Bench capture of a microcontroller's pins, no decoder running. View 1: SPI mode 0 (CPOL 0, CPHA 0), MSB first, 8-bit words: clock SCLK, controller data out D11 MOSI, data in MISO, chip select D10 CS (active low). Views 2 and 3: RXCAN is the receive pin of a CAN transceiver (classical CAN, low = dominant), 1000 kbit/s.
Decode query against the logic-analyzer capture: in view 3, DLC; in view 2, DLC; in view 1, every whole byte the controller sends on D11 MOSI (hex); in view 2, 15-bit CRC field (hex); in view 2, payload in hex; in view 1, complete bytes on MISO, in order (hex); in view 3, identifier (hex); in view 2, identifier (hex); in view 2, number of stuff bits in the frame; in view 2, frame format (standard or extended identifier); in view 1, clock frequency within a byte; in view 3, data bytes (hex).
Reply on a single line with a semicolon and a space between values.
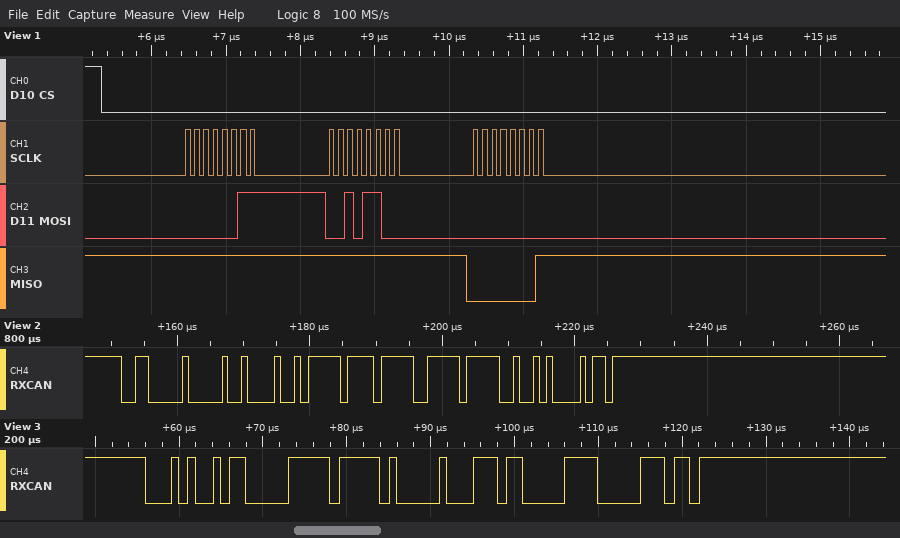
3; 4; 03 2C 00; 0x5285; 25 FF 7D FF; FF FF 01; 0x14B; 0x300; 6; standard; 8 MHz; FF 00 EC
